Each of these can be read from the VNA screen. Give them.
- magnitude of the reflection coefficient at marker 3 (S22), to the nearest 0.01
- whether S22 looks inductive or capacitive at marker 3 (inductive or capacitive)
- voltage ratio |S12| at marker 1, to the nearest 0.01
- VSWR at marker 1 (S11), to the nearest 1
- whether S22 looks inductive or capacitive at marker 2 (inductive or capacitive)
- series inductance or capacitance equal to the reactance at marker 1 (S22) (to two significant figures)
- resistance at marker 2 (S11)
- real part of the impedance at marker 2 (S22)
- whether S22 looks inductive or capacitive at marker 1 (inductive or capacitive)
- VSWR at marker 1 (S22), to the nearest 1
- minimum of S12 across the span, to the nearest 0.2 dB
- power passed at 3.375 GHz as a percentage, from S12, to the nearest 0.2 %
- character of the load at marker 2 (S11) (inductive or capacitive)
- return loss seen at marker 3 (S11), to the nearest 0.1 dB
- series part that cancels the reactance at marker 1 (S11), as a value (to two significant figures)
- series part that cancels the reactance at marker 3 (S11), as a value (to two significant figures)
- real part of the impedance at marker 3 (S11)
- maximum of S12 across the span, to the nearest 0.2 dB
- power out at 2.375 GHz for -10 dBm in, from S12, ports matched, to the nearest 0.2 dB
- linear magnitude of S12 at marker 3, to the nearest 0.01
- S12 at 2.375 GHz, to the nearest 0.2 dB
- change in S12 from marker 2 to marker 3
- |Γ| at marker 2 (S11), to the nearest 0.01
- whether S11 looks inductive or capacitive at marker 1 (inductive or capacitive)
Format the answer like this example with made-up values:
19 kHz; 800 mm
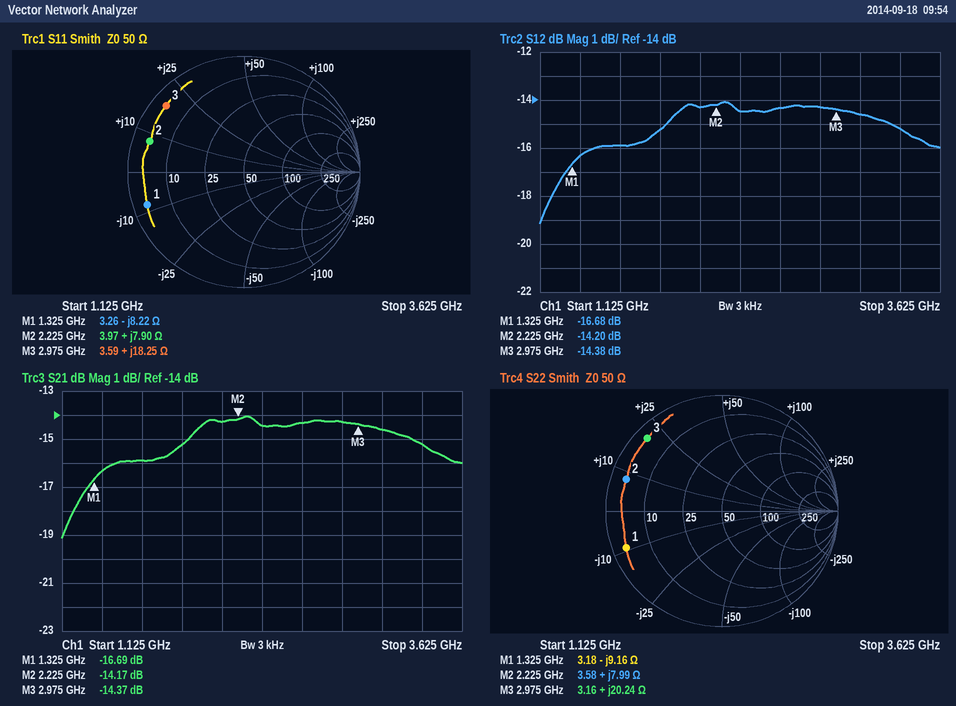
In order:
0.90; inductive; 0.15; 16; inductive; 13 pF; 3.97 Ω; 3.58 Ω; capacitive; 16; -19.2 dB; 3.0 %; inductive; 1.1 dB; 990 pH; 2.9 pF; 3.59 Ω; -14.0 dB; -24.4 dBm; 0.19; -14.4 dB; -0.18 dB; 0.86; capacitive
